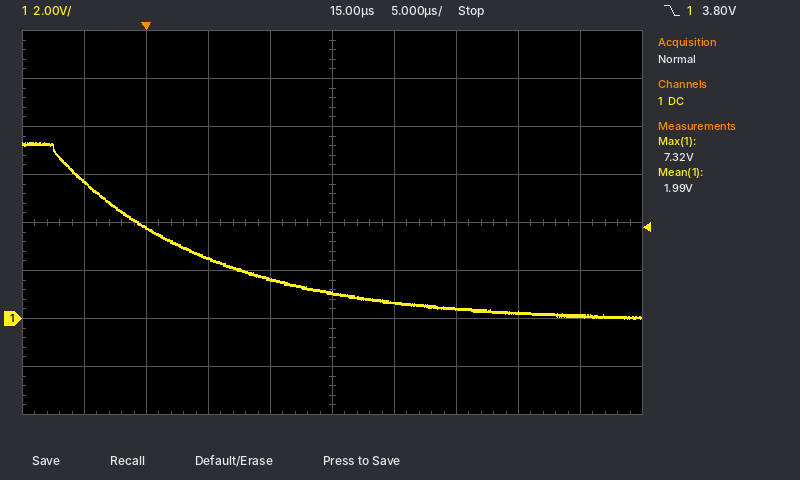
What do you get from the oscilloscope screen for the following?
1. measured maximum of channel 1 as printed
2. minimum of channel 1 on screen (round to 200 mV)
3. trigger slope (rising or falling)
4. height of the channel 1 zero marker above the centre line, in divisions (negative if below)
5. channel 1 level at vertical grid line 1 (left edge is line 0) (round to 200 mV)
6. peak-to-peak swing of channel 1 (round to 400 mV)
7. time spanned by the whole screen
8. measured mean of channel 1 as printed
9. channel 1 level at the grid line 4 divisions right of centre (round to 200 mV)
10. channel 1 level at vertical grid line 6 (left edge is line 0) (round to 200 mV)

7.32 V
0.0 V
falling
-2.0 div
5.8 V
7.2 V
50 µs
1.99 V
200 mV
600 mV
